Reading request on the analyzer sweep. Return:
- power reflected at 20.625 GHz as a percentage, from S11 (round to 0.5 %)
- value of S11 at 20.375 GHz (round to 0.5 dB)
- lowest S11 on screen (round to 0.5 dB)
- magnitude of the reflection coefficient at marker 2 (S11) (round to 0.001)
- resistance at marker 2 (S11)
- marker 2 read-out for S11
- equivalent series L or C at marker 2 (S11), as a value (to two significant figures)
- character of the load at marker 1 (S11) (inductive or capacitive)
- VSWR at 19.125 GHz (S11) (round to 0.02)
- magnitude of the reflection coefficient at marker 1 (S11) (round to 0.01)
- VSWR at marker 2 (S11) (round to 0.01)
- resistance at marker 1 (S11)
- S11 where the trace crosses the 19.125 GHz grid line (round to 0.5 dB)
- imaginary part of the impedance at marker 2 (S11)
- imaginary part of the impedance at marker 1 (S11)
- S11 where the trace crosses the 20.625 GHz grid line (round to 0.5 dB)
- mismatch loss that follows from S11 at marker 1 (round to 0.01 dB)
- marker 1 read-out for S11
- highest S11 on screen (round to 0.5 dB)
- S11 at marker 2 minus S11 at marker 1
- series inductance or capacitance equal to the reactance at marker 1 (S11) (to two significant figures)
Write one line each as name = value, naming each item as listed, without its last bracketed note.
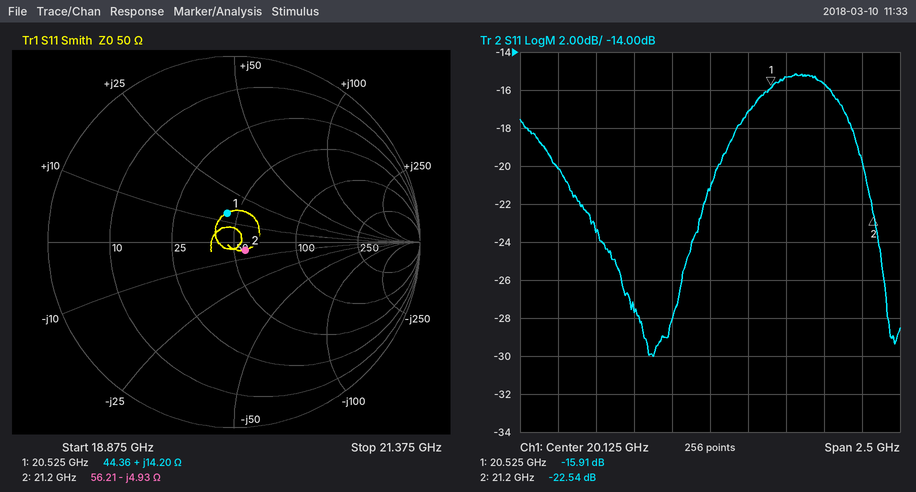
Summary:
power reflected at 20.625 GHz as a percentage, from S11 = 3.0 %
value of S11 at 20.375 GHz = -17.0 dB
lowest S11 on screen = -30.0 dB
magnitude of the reflection coefficient at marker 2 (S11) = 0.075
resistance at marker 2 = 56.21 Ω
marker 2 read-out for S11 = -22.54 dB
equivalent series L or C at marker 2 (S11), as a value = 1.5 pF
character of the load at marker 1 (S11) = inductive
VSWR at 19.125 GHz (S11) = 1.22
magnitude of the reflection coefficient at marker 1 (S11) = 0.16
VSWR at marker 2 (S11) = 1.16
resistance at marker 1 = 44.36 Ω
S11 where the trace crosses the 19.125 GHz grid line = -20.0 dB
imaginary part of the impedance at marker 2 = -4.93 Ω
imaginary part of the impedance at marker 1 = +14.20 Ω
S11 where the trace crosses the 20.625 GHz grid line = -15.5 dB
mismatch loss that follows from S11 at marker 1 = 0.11 dB
marker 1 read-out for S11 = -15.91 dB
highest S11 on screen = -15.0 dB
S11 at marker 2 minus S11 at marker 1 = -6.63 dB
series inductance or capacitance equal to the reactance at marker 1 (S11) = 110 pH
